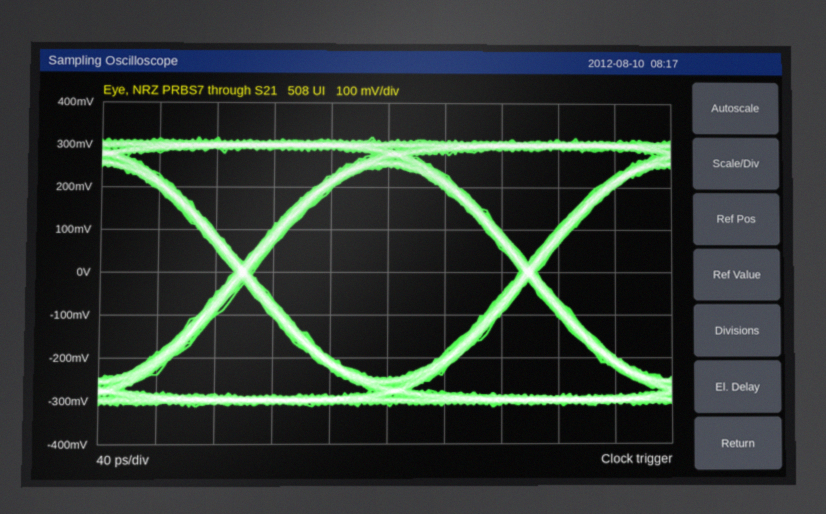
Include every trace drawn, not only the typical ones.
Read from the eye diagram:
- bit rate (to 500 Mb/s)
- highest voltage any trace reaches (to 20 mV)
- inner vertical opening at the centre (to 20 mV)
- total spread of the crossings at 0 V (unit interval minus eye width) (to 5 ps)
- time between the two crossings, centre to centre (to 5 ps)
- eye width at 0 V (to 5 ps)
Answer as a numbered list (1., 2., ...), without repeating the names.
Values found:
1. 5.0 Gb/s
2. 320 mV
3. 500 mV
4. 15 ps
5. 200 ps
6. 185 ps
